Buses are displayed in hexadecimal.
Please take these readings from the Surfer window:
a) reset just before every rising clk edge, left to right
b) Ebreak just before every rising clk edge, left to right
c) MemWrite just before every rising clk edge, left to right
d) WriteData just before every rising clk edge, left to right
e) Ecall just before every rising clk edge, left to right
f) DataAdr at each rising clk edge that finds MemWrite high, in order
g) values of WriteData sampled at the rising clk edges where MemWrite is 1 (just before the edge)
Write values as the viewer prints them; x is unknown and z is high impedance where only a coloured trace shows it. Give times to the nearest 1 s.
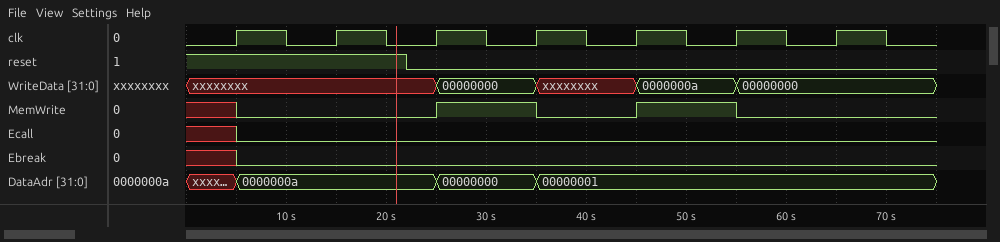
1 1 0 0 0 0 0
x 0 0 0 0 0 0
x 0 0 1 0 1 0
xxxxxxxx, xxxxxxxx, xxxxxxxx, 00000000, xxxxxxxx, 0000000a, 00000000
x 0 0 0 0 0 0
00000000, 00000001
00000000, 0000000a
